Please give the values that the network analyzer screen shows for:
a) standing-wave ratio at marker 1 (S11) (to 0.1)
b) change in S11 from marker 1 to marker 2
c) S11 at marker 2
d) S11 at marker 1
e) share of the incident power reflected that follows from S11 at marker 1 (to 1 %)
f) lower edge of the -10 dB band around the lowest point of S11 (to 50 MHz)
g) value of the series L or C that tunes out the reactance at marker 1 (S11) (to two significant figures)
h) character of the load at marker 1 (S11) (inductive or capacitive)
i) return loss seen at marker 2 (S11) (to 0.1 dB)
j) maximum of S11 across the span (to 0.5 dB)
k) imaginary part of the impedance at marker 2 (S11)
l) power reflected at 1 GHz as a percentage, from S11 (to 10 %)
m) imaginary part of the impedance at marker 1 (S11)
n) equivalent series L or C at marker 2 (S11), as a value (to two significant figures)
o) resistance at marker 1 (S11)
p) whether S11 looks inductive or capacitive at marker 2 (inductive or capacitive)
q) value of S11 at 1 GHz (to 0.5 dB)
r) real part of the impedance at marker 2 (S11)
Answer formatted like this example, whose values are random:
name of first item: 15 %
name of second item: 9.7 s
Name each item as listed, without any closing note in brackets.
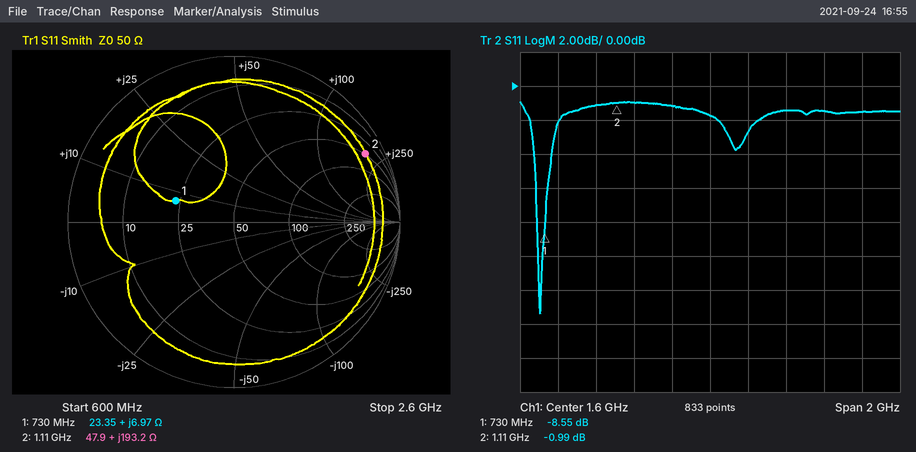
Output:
standing-wave ratio at marker 1 (S11): 2.2
change in S11 from marker 1 to marker 2: 7.56 dB
S11 at marker 2: -0.99 dB
S11 at marker 1: -8.55 dB
share of the incident power reflected that follows from S11 at marker 1: 14 %
lower edge of the -10 dB band around the lowest point of S11: 700 MHz
value of the series L or C that tunes out the reactance at marker 1 (S11): 31 pF
character of the load at marker 1 (S11): inductive
return loss seen at marker 2 (S11): 1.0 dB
maximum of S11 across the span: -1.0 dB
imaginary part of the impedance at marker 2: +193.2 Ω
power reflected at 1 GHz as a percentage, from S11: 80 %
imaginary part of the impedance at marker 1: +6.97 Ω
equivalent series L or C at marker 2 (S11), as a value: 28 nH
resistance at marker 1: 23.35 Ω
whether S11 looks inductive or capacitive at marker 2: inductive
value of S11 at 1 GHz: -1.0 dB
real part of the impedance at marker 2: 47.9 Ω
